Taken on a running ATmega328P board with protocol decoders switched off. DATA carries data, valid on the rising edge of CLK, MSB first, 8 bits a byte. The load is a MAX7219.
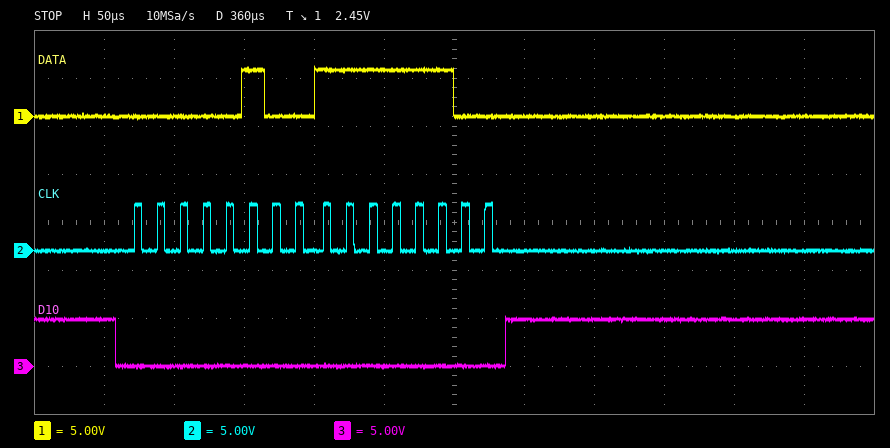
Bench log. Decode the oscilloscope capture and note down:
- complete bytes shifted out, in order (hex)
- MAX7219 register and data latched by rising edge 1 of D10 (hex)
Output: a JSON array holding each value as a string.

["04 FC", "register 0x4, data 0xFC"]
